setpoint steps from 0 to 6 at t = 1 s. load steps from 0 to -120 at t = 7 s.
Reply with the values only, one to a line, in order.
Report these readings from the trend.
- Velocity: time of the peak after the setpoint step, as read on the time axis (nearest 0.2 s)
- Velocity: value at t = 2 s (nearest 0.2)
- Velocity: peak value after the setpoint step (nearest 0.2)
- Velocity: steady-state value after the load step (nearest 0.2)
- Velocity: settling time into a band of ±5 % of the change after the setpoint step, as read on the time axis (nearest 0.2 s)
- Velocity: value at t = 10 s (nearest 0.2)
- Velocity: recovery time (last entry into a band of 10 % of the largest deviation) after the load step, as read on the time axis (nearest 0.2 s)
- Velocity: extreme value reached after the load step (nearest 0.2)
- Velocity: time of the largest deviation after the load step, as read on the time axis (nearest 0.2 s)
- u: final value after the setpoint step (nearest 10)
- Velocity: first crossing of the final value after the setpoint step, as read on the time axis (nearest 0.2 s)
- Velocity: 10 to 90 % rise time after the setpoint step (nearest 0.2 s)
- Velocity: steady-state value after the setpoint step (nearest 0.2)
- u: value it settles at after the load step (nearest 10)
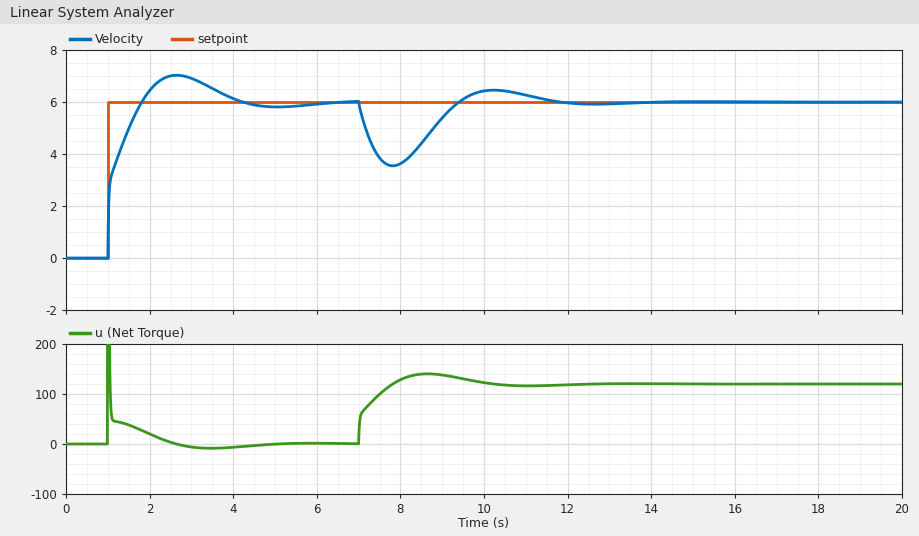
2.6 s
6.4
7.0
6.0
3.8 s
6.4
11.0 s
3.6
7.8 s
0
1.8 s
0.6 s
6.0
120
